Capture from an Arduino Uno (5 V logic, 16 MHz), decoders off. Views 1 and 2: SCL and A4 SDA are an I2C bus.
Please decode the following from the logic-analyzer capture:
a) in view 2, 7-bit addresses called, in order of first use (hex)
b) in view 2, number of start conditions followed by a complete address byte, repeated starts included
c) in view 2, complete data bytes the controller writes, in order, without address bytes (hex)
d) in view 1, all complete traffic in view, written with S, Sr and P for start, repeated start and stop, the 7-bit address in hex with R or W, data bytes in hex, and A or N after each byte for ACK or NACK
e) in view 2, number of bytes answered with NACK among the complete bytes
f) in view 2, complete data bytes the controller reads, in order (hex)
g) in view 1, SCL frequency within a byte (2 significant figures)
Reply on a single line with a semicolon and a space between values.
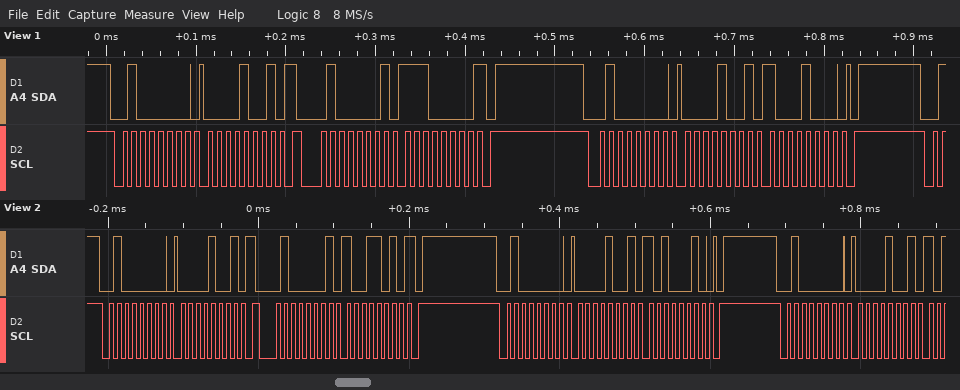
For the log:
0x20; 4; 09 09 A2 09; S 20W A 09 A Sr 20R A E0 N P S 20W A 09 A 88 A P; 1; 9A; 100 kHz
